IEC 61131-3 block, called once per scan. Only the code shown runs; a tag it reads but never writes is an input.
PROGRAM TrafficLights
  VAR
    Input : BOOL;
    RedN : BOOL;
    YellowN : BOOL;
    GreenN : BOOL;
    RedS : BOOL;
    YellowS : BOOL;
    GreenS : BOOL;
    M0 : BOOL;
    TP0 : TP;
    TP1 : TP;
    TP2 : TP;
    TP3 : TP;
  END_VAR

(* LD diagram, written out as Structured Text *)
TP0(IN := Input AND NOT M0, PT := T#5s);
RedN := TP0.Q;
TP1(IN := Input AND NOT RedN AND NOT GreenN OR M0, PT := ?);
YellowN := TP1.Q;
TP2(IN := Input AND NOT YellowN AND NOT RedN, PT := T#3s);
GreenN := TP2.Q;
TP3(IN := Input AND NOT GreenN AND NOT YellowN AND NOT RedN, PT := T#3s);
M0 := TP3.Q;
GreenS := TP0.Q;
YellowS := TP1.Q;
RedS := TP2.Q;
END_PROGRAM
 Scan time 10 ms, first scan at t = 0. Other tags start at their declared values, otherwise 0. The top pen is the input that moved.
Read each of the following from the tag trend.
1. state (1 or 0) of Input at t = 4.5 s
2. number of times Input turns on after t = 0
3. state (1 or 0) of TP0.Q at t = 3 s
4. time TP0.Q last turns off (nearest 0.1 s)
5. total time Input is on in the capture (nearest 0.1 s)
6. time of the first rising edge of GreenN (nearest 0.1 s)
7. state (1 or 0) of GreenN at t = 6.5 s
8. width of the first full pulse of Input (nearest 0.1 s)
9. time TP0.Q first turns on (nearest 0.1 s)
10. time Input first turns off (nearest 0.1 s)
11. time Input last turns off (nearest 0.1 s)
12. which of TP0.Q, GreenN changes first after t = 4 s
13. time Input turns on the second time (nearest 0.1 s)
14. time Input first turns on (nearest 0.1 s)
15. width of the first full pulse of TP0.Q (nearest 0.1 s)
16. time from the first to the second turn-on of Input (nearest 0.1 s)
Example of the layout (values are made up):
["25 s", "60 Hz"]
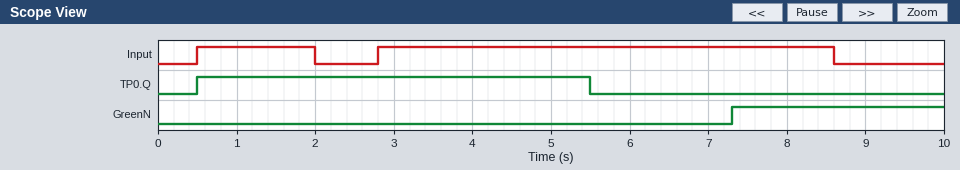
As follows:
["1", "2", "1", "5.5 s", "7.3 s", "7.3 s", "0", "1.5 s", "0.5 s", "2.0 s", "8.6 s", "TP0.Q", "2.8 s", "0.5 s", "5.0 s", "2.3 s"]
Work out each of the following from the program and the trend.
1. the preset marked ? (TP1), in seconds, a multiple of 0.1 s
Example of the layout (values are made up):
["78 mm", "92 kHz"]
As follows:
["1.8 s"]
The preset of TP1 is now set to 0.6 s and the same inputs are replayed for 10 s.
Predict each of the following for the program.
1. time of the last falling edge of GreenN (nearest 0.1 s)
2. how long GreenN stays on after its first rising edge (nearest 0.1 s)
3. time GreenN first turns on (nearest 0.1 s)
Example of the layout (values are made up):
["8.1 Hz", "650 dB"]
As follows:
["9.1 s", "3.0 s", "6.1 s"]
